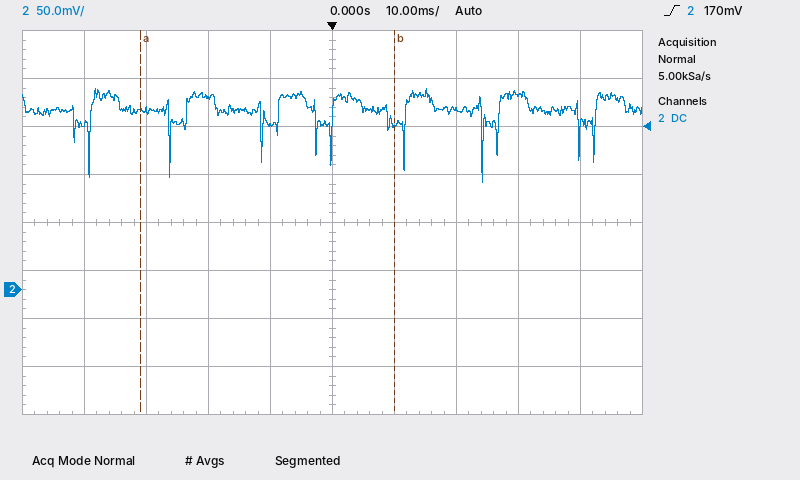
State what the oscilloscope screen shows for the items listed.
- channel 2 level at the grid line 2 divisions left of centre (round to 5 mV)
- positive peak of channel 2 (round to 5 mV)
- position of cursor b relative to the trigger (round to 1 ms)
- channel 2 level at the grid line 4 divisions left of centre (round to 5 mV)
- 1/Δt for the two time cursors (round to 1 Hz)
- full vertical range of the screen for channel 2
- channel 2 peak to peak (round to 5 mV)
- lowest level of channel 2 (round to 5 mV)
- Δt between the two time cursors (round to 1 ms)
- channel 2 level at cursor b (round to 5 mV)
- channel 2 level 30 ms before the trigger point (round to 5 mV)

200 mV
210 mV
+10 ms
175 mV
24 Hz
400 mV
100 mV
110 mV
41 ms
175 mV
185 mV
